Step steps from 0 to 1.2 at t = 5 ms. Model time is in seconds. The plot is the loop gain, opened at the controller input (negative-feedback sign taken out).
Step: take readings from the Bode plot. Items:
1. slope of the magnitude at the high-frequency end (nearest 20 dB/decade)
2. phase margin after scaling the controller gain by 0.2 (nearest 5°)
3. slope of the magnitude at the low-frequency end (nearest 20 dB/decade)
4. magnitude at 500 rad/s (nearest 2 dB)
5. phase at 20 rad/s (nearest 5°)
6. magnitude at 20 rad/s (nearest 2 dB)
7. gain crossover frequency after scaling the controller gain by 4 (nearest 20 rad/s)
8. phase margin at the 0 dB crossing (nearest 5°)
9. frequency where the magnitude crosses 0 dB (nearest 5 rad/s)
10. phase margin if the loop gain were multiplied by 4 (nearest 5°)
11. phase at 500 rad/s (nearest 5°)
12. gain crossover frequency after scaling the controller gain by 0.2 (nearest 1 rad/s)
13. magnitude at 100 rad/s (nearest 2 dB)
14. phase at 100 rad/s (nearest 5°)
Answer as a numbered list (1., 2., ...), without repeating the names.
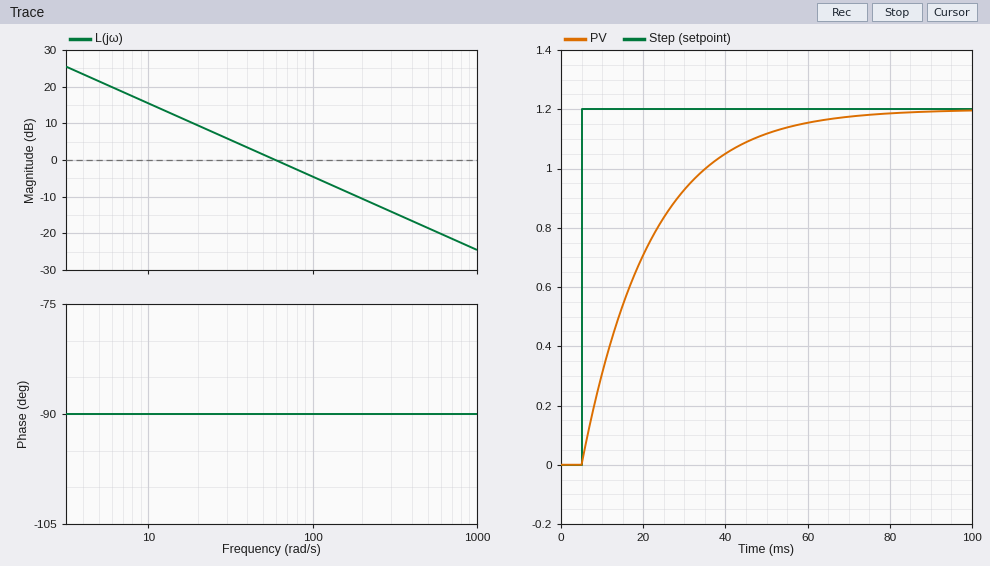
1. -20 dB/decade
2. 90°
3. -20 dB/decade
4. -18 dB
5. -90°
6. 10 dB
7. 240 rad/s
8. 90°
9. 60 rad/s
10. 90°
11. -90°
12. 12 rad/s
13. -4 dB
14. -90°
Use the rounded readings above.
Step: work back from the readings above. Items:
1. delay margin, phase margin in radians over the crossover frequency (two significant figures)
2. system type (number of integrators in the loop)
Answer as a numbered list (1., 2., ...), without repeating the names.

1. 0.026 s
2. 1
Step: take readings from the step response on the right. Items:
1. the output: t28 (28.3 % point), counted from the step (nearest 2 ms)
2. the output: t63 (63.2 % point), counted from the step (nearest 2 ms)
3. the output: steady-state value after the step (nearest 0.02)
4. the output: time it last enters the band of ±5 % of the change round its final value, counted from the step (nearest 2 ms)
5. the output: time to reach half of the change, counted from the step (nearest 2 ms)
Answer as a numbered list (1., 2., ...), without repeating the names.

1. 6 ms
2. 16 ms
3. 1.20
4. 50 ms
5. 12 ms
